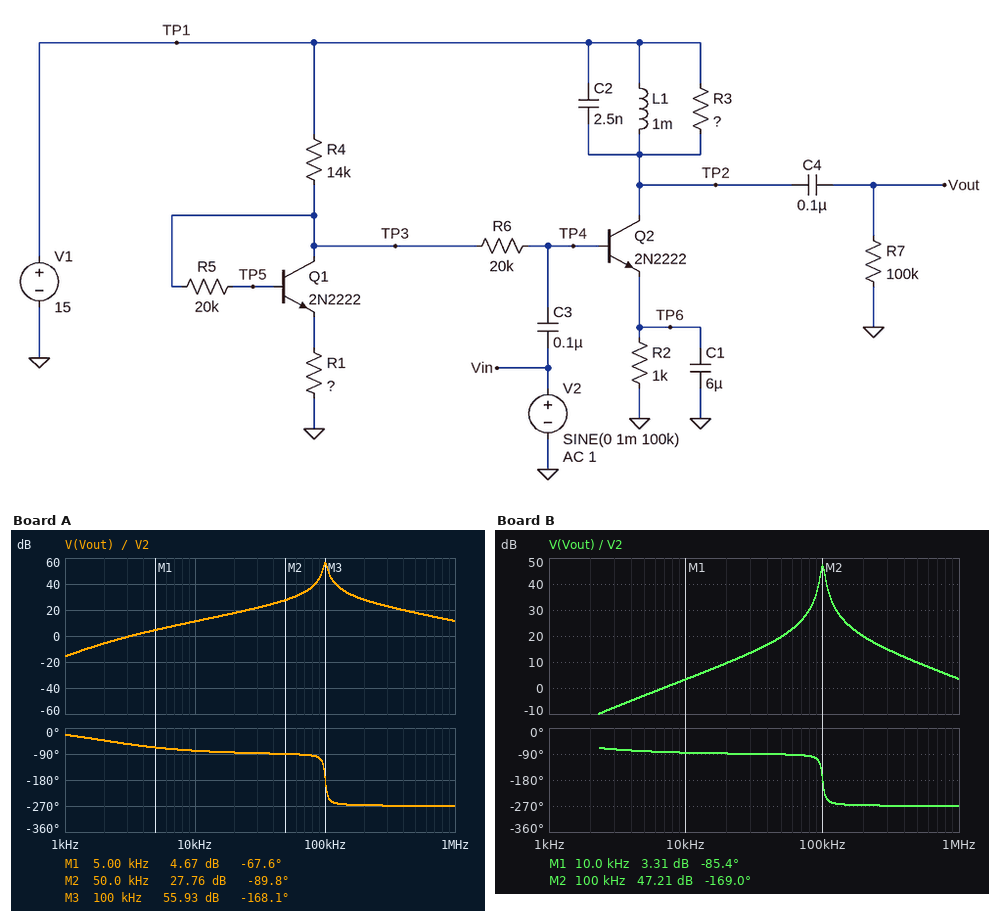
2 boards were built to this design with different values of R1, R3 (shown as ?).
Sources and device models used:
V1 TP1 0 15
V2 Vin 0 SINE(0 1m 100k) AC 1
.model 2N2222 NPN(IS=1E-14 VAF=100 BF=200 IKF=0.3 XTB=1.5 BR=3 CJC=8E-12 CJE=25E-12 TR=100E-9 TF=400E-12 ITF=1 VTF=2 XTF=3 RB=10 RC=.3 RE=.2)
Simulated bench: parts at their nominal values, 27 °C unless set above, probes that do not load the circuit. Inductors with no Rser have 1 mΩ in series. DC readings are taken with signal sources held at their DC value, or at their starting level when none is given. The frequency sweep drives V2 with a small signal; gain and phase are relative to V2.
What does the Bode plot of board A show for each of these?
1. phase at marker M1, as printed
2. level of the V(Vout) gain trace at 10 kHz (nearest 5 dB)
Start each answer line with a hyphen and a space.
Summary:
- -67.6 deg
- 10 dB
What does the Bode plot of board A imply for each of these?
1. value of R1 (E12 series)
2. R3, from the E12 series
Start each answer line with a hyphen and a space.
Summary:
- 1.8 kΩ
- 15 kΩ
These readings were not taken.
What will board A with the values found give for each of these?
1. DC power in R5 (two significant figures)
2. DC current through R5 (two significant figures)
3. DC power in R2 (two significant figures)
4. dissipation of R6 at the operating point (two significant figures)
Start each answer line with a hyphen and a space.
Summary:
- 400 nW
- 4.5 µA
- 2.4 mW
- 950 nW
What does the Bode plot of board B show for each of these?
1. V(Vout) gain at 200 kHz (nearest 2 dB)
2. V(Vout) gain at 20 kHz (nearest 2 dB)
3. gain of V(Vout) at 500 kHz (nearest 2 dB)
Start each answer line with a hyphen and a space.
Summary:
- 20 dB
- 10 dB
- 10 dB
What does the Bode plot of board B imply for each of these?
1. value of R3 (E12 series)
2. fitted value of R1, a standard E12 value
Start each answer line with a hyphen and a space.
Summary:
- 12 kΩ
- 560 Ω
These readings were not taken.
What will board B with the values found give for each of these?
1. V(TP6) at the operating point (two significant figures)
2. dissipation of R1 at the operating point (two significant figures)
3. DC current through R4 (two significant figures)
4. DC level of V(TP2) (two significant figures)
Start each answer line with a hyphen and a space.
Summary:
- 610 mV
- 530 µW
- 980 µA
- 15 V
